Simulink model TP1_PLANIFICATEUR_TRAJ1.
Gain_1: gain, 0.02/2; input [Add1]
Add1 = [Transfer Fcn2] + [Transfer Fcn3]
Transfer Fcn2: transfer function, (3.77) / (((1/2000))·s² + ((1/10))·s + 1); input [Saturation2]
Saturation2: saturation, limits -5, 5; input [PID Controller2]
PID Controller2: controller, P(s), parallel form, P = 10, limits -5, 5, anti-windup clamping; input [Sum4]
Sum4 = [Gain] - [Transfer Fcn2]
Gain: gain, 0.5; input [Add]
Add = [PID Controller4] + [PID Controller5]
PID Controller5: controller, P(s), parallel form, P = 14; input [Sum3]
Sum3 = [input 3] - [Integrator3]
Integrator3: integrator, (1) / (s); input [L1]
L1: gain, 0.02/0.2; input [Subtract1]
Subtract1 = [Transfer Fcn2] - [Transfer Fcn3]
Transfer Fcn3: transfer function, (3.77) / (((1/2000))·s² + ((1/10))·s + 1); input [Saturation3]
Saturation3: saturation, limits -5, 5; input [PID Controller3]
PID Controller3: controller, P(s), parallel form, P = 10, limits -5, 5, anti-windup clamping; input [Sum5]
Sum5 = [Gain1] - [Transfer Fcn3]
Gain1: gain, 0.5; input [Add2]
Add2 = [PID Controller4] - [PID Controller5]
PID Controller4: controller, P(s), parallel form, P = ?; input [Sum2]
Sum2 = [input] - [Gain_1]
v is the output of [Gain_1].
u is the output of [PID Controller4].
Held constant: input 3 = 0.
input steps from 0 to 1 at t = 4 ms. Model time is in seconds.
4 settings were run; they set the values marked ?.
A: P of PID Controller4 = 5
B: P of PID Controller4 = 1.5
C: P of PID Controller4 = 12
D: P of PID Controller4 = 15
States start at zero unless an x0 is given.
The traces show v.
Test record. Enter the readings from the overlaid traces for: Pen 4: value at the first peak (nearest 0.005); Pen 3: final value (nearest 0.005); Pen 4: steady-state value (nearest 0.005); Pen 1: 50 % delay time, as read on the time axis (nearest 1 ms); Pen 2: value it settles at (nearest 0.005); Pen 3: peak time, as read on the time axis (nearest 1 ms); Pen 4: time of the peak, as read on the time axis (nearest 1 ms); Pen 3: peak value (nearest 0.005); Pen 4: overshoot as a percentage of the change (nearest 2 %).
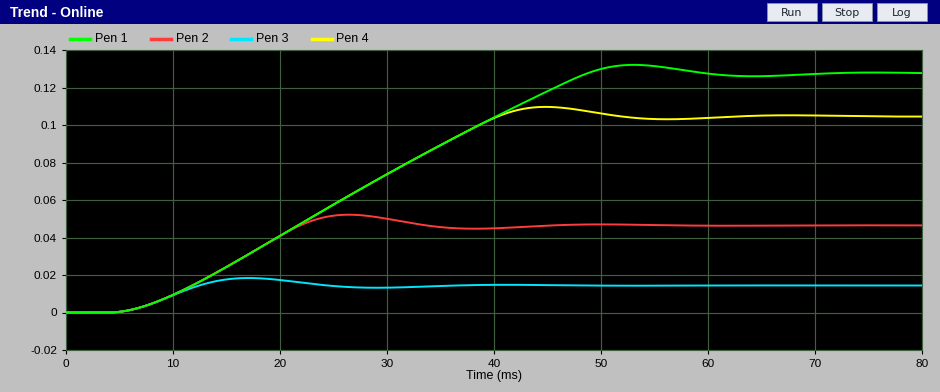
0.110
0.015
0.105
27 ms
0.045
17 ms
45 ms
0.020
4 %
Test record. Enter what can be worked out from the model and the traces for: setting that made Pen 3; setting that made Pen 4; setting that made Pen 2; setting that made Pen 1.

B
C
A
D
